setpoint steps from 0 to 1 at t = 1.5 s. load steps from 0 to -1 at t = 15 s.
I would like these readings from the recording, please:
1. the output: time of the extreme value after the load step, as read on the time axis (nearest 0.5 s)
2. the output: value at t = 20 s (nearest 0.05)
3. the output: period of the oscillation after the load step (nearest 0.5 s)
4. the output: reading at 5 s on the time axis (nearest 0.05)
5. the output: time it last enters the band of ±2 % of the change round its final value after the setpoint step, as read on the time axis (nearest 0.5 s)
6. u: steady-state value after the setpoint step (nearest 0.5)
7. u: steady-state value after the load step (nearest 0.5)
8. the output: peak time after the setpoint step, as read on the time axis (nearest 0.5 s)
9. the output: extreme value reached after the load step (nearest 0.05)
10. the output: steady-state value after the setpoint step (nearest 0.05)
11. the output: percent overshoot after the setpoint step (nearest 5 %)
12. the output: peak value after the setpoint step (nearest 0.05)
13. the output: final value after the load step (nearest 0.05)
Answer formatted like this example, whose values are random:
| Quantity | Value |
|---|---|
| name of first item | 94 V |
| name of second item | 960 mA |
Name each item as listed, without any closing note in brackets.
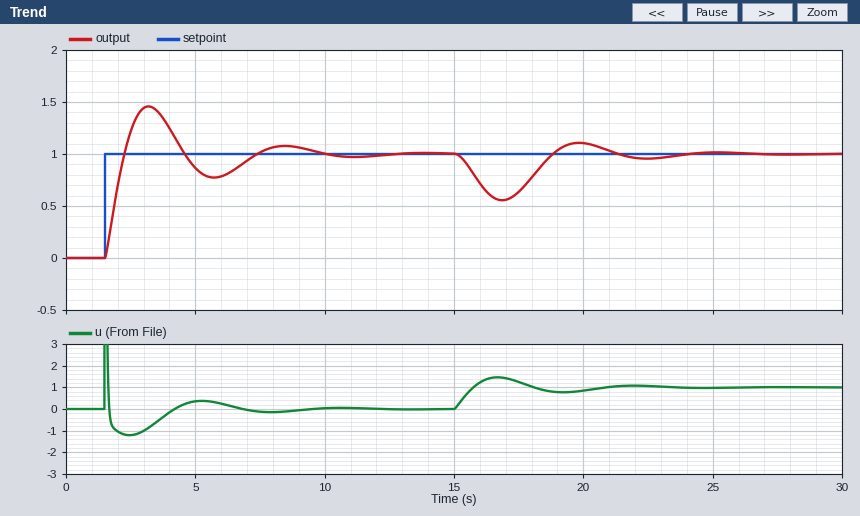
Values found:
| Quantity | Value |
|---|---|
| the output: time of the extreme value after the load step, as read on the time axis | 17.0 s |
| the output: value at t = 20 s | 1.10 |
| the output: period of the oscillation after the load step | 5.5 s |
| the output: reading at 5 s on the time axis | 0.85 |
| the output: time it last enters the band of ±2 % of the change round its final value after the setpoint step, as read on the time axis | 12.0 s |
| u: steady-state value after the setpoint step | 0.0 |
| u: steady-state value after the load step | 1.0 |
| the output: peak time after the setpoint step, as read on the time axis | 3.0 s |
| the output: extreme value reached after the load step | 0.55 |
| the output: steady-state value after the setpoint step | 1.00 |
| the output: percent overshoot after the setpoint step | 45 % |
| the output: peak value after the setpoint step | 1.45 |
| the output: final value after the load step | 1.00 |
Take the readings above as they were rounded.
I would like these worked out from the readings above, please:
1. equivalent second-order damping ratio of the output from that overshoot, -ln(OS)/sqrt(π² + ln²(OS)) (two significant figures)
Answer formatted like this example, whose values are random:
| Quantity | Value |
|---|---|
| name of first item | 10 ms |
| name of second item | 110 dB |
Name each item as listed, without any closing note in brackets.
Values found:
| Quantity | Value |
|---|---|
| equivalent second-order damping ratio of the output from that overshoot, -ln(OS)/sqrt(π² + ln²(OS)) | 0.25 |
